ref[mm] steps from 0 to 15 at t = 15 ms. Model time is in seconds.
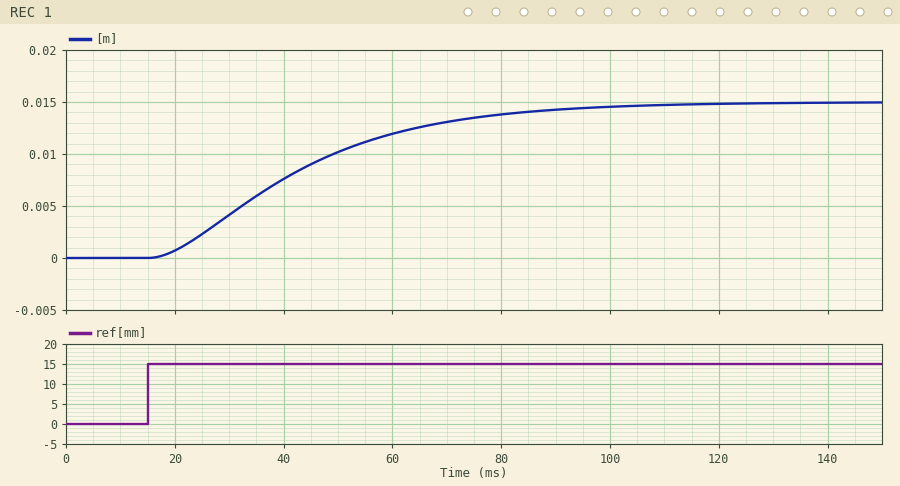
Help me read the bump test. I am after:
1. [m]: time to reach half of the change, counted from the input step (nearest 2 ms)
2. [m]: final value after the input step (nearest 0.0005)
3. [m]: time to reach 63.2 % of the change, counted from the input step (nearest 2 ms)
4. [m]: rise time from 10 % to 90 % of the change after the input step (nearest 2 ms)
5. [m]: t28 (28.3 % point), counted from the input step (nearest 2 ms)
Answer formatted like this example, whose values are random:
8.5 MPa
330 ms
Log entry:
24 ms
0.0150
32 ms
52 ms
16 ms
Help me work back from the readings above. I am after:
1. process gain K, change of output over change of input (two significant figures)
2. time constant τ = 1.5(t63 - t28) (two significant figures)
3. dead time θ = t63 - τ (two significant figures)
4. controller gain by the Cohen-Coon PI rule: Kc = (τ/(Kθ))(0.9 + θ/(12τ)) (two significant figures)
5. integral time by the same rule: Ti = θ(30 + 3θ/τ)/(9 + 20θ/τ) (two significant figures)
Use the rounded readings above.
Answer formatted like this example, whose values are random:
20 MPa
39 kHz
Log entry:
0.0010
24 ms
8.0 ms
2800
16 ms
